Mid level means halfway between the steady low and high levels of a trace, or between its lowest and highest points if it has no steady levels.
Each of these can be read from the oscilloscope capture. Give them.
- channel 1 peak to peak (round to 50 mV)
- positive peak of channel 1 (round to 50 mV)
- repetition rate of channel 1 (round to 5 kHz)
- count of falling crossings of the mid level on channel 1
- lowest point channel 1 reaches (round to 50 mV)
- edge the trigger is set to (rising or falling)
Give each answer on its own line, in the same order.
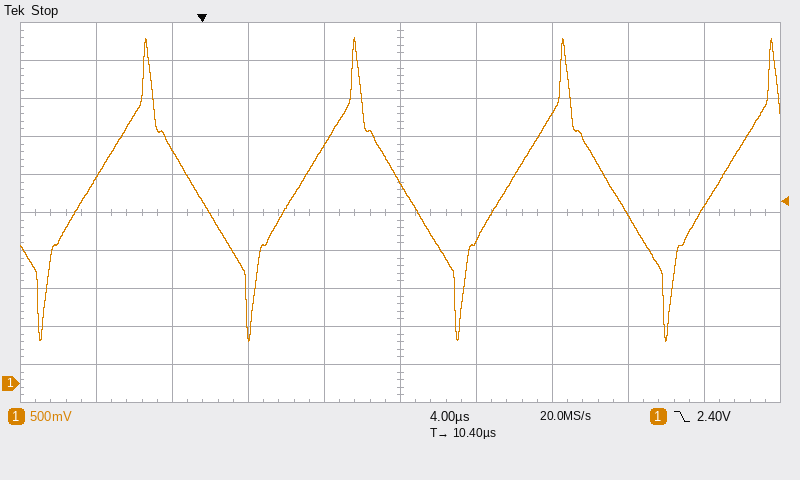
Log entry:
4.00 V
4.55 V
90 kHz
3
550 mV
falling
